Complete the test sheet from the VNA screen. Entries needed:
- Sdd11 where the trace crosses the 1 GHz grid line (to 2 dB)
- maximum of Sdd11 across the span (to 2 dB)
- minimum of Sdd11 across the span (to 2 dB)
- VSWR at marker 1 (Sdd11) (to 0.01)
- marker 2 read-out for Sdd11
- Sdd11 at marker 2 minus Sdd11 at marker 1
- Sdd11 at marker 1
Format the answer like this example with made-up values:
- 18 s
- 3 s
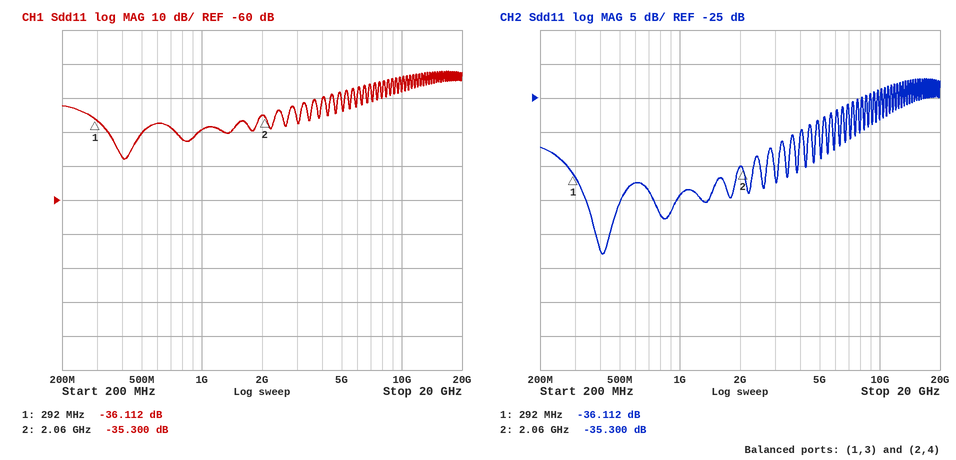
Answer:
- -40 dB
- -22 dB
- -48 dB
- 1.03
- -35.300 dB
- 0.812 dB
- -36.112 dB
